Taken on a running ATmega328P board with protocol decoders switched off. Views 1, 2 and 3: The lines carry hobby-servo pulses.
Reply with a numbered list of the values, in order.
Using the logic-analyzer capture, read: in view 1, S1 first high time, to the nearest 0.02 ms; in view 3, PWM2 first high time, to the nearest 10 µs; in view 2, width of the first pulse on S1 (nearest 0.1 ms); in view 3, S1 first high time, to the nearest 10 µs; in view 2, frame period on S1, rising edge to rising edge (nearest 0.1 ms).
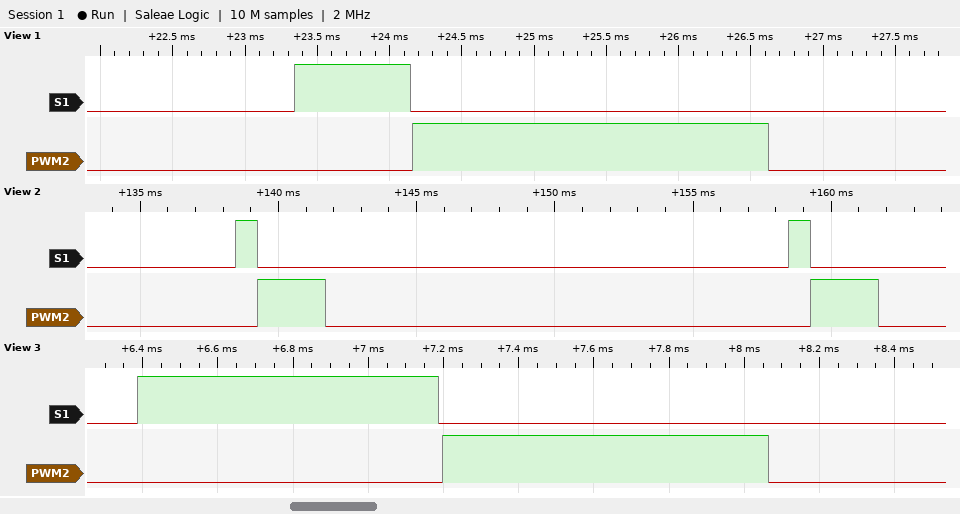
1. 0.80 ms
2. 870 µs
3. 0.8 ms
4. 800 µs
5. 20.0 ms
